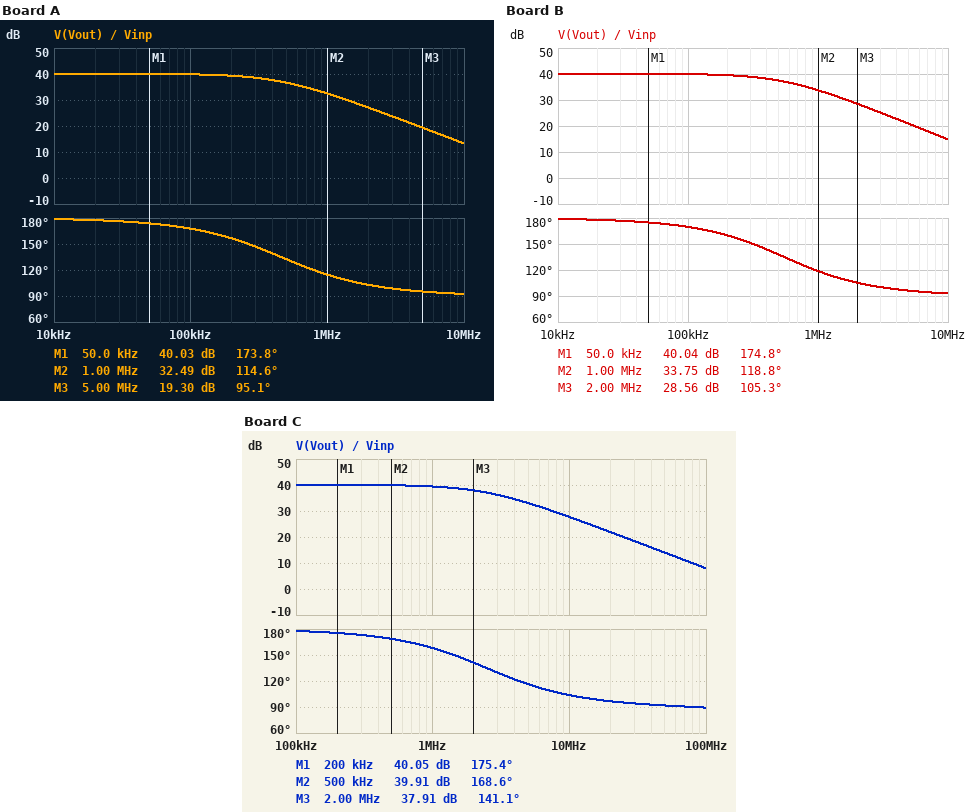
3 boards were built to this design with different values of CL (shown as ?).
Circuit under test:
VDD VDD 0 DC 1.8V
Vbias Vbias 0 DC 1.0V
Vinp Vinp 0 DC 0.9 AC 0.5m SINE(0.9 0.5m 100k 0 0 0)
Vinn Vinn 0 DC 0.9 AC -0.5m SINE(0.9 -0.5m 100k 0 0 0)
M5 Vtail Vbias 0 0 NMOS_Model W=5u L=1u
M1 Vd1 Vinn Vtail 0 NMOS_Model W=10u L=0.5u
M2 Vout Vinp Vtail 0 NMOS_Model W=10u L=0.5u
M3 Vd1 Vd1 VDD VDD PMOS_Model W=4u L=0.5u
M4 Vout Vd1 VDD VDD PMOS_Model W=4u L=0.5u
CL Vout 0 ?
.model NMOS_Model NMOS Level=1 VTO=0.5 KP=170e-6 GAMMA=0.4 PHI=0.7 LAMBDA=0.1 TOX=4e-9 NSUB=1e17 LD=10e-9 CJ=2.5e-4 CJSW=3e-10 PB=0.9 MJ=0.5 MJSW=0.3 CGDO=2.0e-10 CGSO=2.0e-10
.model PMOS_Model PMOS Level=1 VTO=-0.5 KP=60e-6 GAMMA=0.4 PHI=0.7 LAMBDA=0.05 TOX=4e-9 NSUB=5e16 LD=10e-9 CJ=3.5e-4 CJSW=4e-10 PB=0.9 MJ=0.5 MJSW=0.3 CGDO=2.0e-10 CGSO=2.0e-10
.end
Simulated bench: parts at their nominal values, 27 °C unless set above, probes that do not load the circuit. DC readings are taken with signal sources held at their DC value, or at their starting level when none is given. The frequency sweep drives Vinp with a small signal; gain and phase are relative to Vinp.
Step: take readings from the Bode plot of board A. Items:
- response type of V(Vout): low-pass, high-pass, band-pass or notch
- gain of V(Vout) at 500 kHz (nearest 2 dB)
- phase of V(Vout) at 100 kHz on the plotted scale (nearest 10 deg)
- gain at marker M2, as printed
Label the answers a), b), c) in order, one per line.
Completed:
a) low-pass
b) 36 dB
c) 170 deg
d) 32.49 dB
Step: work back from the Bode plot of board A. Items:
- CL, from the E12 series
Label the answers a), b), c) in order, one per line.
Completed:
a) 1.8 pF
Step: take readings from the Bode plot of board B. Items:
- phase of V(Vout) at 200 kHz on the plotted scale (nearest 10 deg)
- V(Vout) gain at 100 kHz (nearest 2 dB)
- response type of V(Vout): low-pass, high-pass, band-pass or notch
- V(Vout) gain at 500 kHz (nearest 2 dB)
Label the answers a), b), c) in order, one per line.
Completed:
a) 160 deg
b) 40 dB
c) low-pass
d) 38 dB
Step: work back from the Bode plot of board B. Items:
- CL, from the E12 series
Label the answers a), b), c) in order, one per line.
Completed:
a) 1.5 pF
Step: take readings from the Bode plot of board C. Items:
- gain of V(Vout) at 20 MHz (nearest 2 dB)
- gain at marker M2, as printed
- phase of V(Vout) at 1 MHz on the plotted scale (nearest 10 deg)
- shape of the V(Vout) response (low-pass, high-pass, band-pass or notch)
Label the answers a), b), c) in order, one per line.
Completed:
a) 22 dB
b) 39.91 dB
c) 160 deg
d) low-pass
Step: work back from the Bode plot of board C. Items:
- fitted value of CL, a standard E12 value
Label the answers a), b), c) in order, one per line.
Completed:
a) 330 fF
